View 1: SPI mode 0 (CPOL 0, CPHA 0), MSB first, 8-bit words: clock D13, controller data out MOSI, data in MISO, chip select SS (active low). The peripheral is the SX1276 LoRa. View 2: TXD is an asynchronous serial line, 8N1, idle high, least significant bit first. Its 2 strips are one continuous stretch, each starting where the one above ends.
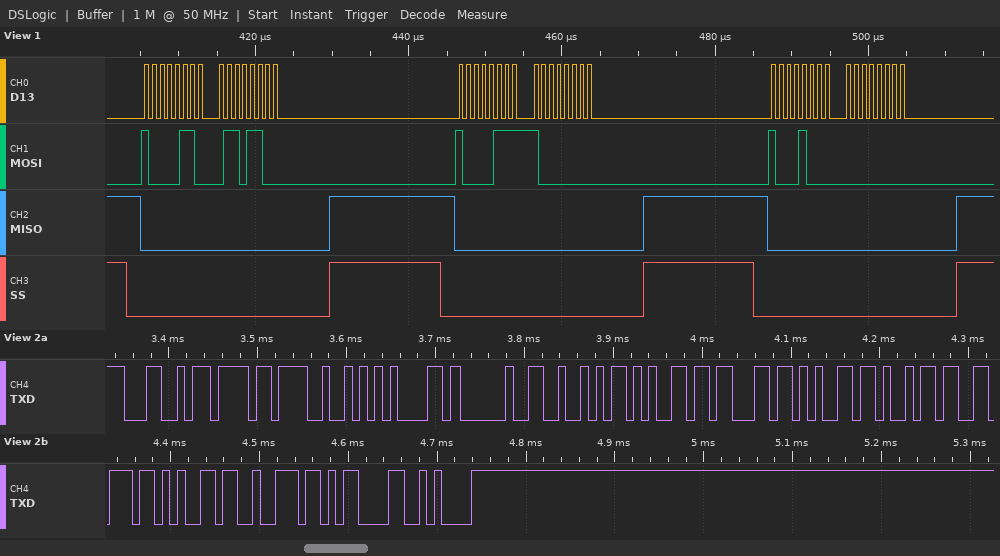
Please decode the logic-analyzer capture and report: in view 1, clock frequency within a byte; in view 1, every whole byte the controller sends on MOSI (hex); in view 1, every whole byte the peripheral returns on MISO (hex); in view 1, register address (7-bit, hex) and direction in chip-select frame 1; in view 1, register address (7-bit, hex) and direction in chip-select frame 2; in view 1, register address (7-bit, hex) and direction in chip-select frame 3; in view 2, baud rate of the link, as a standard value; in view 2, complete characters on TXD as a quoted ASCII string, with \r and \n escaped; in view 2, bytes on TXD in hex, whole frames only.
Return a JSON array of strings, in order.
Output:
["1 MHz", "86 6C 87 80 88 00", "00 00 00 00 00 00", "0x06 write", "0x07 write", "0x08 write", "115200 baud", "\"LoRa Receiver\\r\\n\"", "0x4C 0x6F 0x52 0x61 0x20 0x52 0x65 0x63 0x65 0x69 0x76 0x65 0x72 0x0D 0x0A"]
